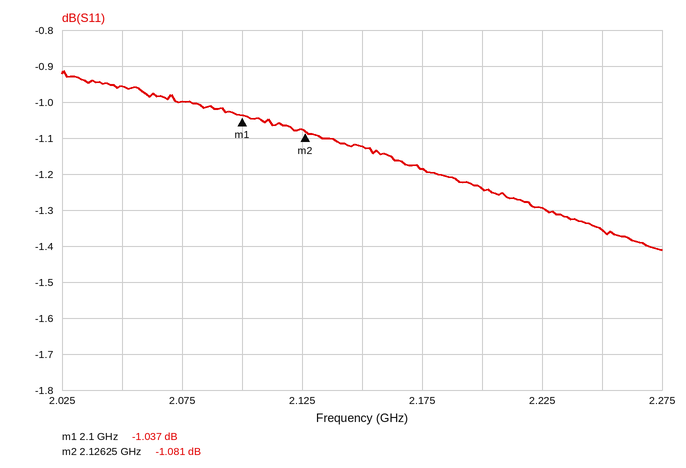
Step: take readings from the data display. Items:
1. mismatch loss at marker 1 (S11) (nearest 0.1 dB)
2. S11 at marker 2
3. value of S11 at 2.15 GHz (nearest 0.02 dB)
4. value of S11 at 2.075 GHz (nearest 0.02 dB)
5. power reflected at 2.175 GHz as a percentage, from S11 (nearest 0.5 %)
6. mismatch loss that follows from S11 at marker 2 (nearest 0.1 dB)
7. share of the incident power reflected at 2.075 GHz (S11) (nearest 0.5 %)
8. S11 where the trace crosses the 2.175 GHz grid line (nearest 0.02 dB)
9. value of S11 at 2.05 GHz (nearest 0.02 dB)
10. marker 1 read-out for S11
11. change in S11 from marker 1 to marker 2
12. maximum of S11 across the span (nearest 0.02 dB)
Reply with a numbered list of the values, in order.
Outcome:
1. 6.7 dB
2. -1.081 dB
3. -1.12 dB
4. -1.00 dB
5. 76.0 %
6. 6.6 dB
7. 79.5 %
8. -1.18 dB
9. -0.96 dB
10. -1.037 dB
11. -0.044 dB
12. -0.92 dB
